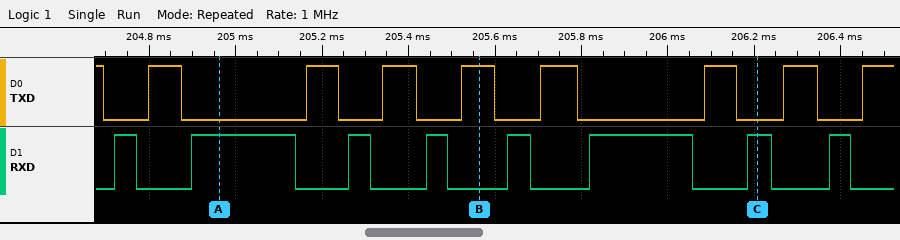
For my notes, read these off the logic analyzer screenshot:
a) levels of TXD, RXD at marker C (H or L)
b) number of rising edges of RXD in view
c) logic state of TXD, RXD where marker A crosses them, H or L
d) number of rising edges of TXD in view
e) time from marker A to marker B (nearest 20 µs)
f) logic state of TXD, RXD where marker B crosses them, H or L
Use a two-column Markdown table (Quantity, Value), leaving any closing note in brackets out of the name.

| Quantity | Value |
|---|---|
| levels of TXD, RXD at marker C | TXD=L, RXD=H |
| number of rising edges of RXD in view | 8 |
| logic state of TXD, RXD where marker A crosses them, H or L | TXD=L, RXD=H |
| number of rising edges of TXD in view | 8 |
| time from marker A to marker B | 600 µs |
| logic state of TXD, RXD where marker B crosses them, H or L | TXD=H, RXD=L |
